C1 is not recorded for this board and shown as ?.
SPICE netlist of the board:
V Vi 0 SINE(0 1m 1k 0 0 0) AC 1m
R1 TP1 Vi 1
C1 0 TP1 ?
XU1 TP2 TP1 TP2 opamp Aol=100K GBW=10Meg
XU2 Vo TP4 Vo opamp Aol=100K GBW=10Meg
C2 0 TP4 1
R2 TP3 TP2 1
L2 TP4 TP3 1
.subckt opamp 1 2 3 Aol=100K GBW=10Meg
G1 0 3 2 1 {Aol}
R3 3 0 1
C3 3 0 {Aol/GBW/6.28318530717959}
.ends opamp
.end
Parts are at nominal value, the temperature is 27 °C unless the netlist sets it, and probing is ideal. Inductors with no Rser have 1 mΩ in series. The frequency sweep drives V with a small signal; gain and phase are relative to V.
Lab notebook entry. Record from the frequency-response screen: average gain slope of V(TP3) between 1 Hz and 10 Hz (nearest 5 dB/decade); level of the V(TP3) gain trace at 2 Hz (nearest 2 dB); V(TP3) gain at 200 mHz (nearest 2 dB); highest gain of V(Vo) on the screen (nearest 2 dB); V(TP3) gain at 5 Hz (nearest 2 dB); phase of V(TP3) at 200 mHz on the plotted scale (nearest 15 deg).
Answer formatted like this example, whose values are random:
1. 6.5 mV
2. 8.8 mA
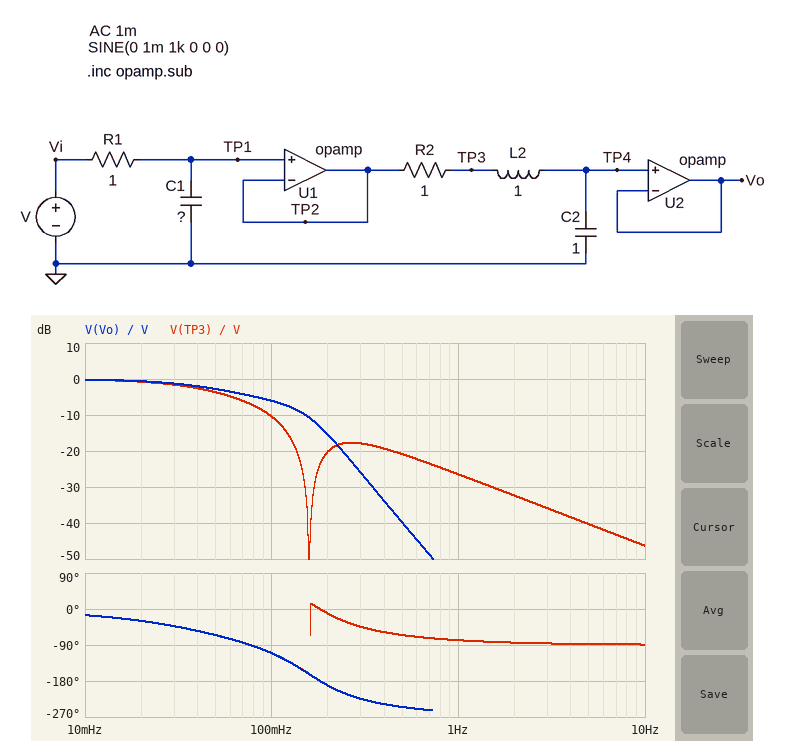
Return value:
1. -20 dB/decade
2. -32 dB
3. -20 dB
4. 0 dB
5. -40 dB
6. -15 deg
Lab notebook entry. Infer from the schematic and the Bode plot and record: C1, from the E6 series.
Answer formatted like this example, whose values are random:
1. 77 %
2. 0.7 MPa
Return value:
1. 3.3 F
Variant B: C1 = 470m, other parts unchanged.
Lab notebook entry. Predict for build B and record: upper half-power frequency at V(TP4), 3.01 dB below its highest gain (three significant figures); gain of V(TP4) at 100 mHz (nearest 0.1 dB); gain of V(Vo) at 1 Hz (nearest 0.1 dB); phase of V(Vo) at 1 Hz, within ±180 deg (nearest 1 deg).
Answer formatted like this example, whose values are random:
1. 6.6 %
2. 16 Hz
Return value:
1. 177 mHz
2. 0.8 dB
3. -41.7 dB
4. 118 deg
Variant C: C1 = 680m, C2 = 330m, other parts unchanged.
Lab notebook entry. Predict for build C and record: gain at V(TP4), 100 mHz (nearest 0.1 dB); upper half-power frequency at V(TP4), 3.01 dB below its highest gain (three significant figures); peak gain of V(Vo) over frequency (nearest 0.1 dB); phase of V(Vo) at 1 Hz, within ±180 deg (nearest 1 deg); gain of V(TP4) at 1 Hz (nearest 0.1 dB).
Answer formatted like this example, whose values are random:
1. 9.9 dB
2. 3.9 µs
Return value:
1. 0.2 dB
2. 308 mHz
3. 2.0 dB
4. 113 deg
5. -34.6 dB
